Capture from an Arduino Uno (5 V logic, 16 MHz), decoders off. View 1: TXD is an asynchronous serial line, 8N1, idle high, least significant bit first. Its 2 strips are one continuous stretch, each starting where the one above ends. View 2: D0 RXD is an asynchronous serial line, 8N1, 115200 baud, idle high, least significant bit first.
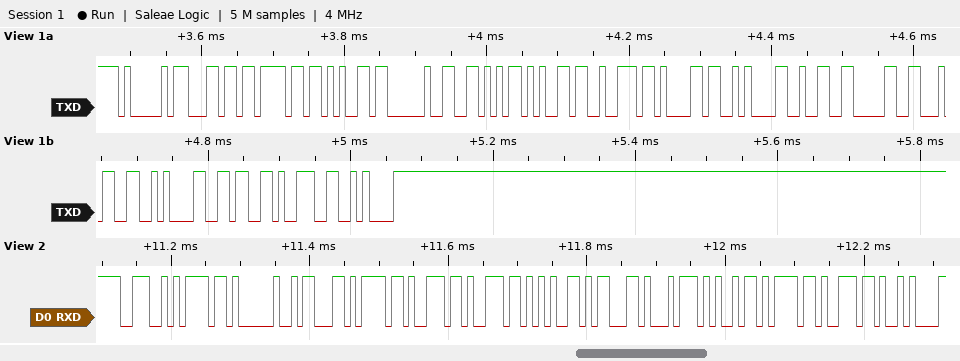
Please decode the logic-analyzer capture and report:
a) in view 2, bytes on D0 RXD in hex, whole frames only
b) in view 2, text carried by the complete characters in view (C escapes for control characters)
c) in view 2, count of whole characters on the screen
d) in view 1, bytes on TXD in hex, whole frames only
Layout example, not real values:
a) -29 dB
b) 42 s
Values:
a) 4E 6F 20 63 6F 6E 6E 65 63 74 69 6F 6E 0A
b) "No connection\n"
c) 14
d) 41 6C 6F 65 20 56 65 72 61 0A 32 30 34 0A 36 39 0A
